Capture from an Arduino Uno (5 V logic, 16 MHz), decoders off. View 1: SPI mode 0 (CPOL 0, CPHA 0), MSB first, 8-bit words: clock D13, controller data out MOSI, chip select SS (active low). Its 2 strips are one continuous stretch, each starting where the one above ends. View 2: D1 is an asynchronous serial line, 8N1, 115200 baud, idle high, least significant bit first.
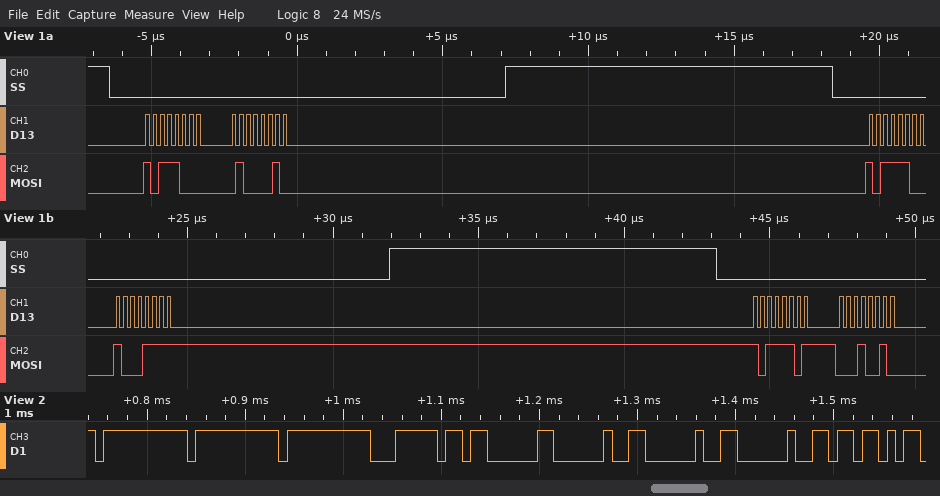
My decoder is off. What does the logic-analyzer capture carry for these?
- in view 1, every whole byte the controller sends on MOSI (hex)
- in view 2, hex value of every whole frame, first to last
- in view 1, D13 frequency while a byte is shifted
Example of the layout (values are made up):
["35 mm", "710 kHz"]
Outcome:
["0xB8 0x42 0xBC 0x8F 0xBD 0x12", "FF FF FF 7C 03 20 20 20 5B", "4 MHz"]
